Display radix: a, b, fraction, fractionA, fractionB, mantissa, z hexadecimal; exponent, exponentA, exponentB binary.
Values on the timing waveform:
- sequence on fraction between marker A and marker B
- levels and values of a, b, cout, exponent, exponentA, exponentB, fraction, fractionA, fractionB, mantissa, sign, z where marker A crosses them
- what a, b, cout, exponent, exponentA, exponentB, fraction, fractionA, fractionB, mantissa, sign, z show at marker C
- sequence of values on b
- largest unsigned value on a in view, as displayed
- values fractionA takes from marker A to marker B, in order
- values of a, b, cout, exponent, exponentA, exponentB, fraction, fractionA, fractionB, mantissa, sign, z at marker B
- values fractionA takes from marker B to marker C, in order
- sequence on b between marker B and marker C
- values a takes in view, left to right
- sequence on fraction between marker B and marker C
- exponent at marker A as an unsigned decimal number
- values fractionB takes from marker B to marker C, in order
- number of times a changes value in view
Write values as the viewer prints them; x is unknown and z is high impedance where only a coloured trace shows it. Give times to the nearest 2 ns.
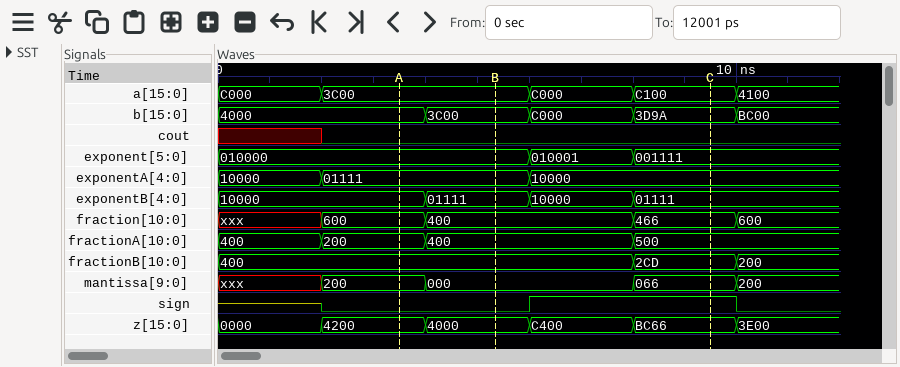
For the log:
600, 400
a=3C00, b=4000, cout=0, exponent=010000, exponentA=01111, exponentB=10000, fraction=600, fractionA=200, fractionB=400, mantissa=200, sign=0, z=4200
a=C100, b=3D9A, cout=0, exponent=001111, exponentA=10000, exponentB=01111, fraction=466, fractionA=500, fractionB=2CD, mantissa=066, sign=1, z=BC66
4000, 3C00, C000, 3D9A, BC00
C100
200, 400
a=3C00, b=3C00, cout=0, exponent=010000, exponentA=01111, exponentB=01111, fraction=400, fractionA=400, fractionB=400, mantissa=000, sign=0, z=4000
400, 500
3C00, C000, 3D9A
C000, 3C00, C000, C100, 4100
400, 466
16
400, 2CD
4
